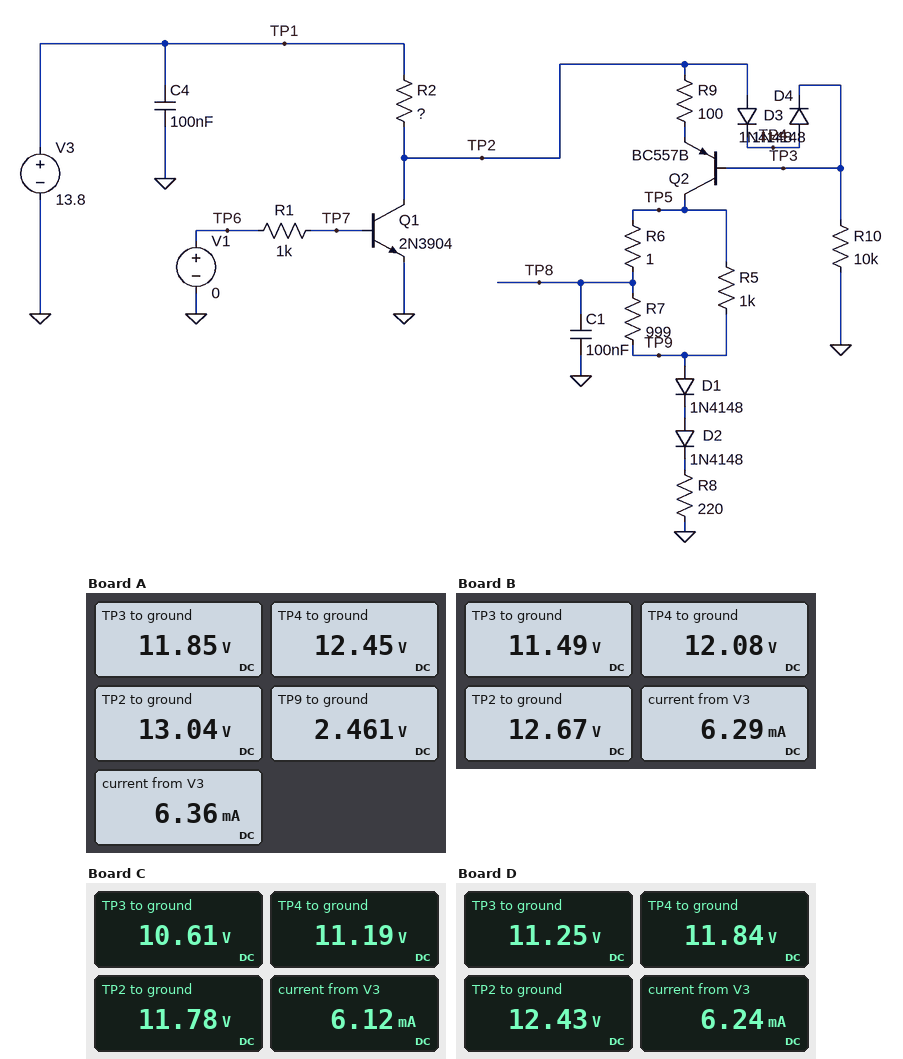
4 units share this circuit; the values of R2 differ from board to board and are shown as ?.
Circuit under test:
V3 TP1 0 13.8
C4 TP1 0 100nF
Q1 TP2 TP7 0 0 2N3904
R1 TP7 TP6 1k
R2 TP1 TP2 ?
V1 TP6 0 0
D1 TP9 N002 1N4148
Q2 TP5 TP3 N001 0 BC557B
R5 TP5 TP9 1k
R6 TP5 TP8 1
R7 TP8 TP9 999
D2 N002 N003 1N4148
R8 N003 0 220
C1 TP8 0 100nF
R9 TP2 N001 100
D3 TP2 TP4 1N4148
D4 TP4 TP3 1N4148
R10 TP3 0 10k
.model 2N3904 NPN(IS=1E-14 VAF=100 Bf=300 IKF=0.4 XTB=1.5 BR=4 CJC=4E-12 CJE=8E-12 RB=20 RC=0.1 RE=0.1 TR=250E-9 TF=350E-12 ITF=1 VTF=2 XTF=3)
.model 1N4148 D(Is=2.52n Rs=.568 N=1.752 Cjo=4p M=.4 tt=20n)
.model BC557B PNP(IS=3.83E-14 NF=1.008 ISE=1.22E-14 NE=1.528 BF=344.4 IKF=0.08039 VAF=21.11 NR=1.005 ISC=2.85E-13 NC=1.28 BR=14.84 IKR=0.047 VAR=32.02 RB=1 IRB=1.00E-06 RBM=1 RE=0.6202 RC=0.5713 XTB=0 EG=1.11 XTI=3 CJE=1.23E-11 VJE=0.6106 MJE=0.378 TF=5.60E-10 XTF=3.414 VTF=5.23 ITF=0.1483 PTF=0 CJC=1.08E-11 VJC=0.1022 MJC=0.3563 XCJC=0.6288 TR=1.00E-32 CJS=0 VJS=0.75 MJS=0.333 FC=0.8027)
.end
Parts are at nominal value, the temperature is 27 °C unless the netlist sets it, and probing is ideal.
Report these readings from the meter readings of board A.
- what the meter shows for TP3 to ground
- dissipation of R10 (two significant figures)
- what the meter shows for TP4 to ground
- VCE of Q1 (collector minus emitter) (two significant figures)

11.85 V
14 mW
12.45 V
13 V
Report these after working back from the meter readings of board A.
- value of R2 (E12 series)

120 Ω
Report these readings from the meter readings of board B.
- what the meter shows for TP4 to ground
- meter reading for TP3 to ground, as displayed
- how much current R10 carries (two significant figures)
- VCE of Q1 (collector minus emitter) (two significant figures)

12.08 V
11.49 V
1.1 mA
13 V
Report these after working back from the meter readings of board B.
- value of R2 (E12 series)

180 Ω
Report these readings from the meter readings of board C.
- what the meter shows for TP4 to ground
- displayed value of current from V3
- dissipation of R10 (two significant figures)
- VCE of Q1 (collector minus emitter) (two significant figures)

11.19 V
6.12 mA
11 mW
12 V
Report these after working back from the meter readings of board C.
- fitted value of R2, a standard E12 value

330 Ω
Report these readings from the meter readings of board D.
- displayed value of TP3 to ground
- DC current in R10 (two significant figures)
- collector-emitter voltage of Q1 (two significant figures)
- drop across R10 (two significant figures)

11.25 V
1.1 mA
12 V
11 V
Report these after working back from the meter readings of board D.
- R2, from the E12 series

220 Ω
